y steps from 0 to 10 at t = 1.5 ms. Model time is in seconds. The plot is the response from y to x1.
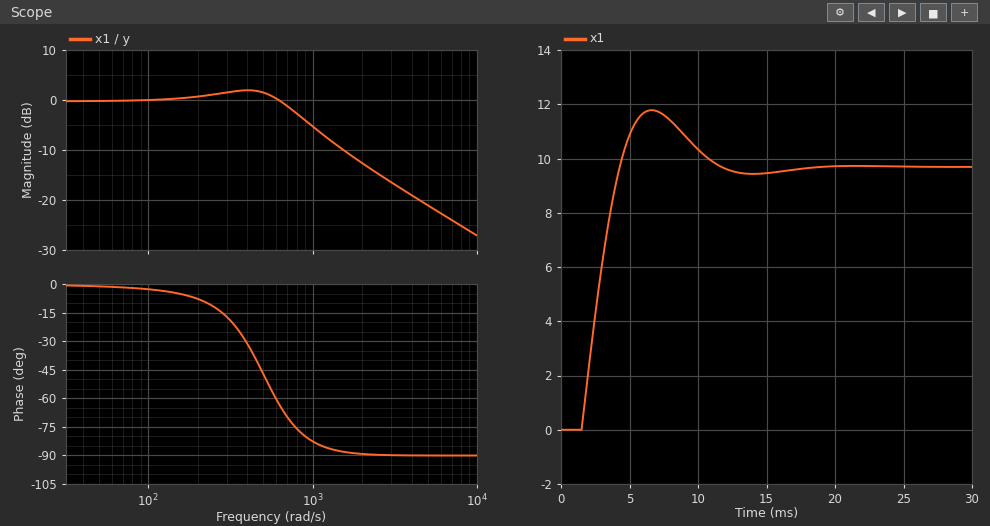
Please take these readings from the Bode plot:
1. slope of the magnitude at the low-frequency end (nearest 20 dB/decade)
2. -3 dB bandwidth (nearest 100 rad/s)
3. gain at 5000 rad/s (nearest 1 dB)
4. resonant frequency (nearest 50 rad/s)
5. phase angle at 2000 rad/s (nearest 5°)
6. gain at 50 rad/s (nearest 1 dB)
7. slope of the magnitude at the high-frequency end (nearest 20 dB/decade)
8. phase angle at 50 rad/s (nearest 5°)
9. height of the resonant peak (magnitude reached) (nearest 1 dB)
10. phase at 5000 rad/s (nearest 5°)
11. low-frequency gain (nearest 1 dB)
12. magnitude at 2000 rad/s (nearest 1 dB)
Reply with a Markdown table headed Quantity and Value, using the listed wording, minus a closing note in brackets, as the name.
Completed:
| Quantity | Value |
|---|---|
| slope of the magnitude at the low-frequency end | 0 dB/decade |
| -3 dB bandwidth | 800 rad/s |
| gain at 5000 rad/s | -21 dB |
| resonant frequency | 400 rad/s |
| phase angle at 2000 rad/s | -90° |
| gain at 50 rad/s | 0 dB |
| slope of the magnitude at the high-frequency end | -20 dB/decade |
| phase angle at 50 rad/s | 0° |
| height of the resonant peak (magnitude reached) | 2 dB |
| phase at 5000 rad/s | -90° |
| low-frequency gain | 0 dB |
| magnitude at 2000 rad/s | -13 dB |
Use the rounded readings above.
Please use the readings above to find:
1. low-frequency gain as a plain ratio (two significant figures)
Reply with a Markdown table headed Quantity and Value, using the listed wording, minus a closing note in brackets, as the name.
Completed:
| Quantity | Value |
|---|---|
| low-frequency gain as a plain ratio | 1.0 |
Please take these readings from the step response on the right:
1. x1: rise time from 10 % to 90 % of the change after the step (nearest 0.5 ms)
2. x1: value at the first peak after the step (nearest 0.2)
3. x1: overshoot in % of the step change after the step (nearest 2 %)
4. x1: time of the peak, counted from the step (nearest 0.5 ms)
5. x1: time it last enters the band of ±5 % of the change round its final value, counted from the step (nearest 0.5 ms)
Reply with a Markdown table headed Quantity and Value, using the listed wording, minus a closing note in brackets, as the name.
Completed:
| Quantity | Value |
|---|---|
| x1: rise time from 10 % to 90 % of the change after the step | 2.0 ms |
| x1: value at the first peak after the step | 11.8 |
| x1: overshoot in % of the step change after the step | 22 % |
| x1: time of the peak, counted from the step | 5.0 ms |
| x1: time it last enters the band of ±5 % of the change round its final value, counted from the step | 9.0 ms |
